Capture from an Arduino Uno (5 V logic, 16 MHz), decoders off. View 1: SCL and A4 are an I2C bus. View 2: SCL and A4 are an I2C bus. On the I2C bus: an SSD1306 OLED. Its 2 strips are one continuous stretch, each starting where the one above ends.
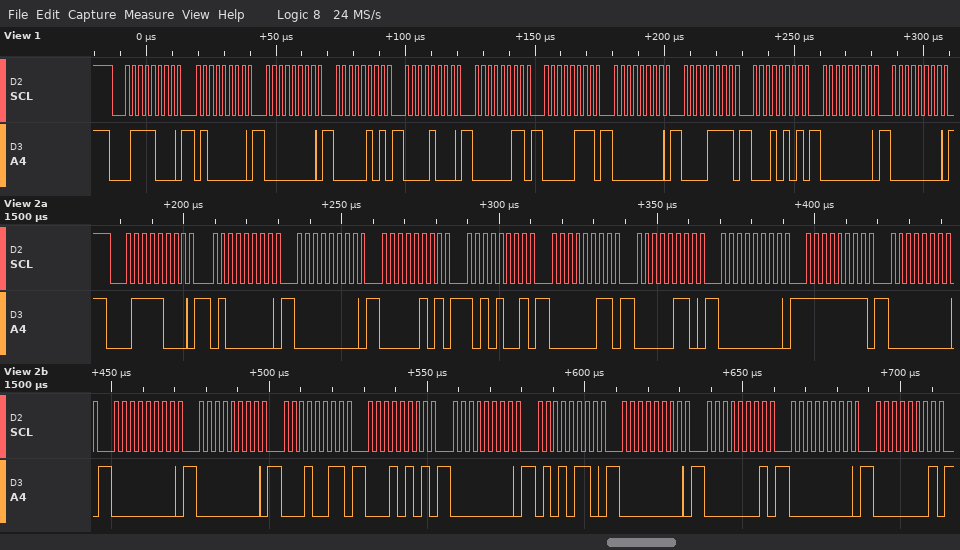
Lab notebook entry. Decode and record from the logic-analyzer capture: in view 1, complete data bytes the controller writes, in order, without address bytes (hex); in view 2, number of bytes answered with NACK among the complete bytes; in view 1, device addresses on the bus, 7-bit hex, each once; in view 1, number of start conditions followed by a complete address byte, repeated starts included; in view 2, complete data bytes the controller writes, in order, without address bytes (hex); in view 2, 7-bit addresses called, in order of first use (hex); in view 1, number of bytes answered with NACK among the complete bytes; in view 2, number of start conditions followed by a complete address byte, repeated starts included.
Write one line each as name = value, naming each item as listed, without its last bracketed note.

in view 1, complete data bytes the controller writes, in order, without address bytes = 40 00 05 08 03 07 00 0F 15 00 00
in view 2, number of bytes answered with NACK among the complete bytes = 0
in view 1, device addresses on the bus, 7-bit hex, each once = 0x3C
in view 1, number of start conditions followed by a complete address byte, repeated starts included = 1
in view 2, complete data bytes the controller writes, in order, without address bytes = 40 00 05 A9 03 06 00 FF 00 00 00 13 15 00 56 00 01 00 01
in view 2, 7-bit addresses called, in order of first use = 0x3C
in view 1, number of bytes answered with NACK among the complete bytes = 0
in view 2, number of start conditions followed by a complete address byte, repeated starts included = 1
